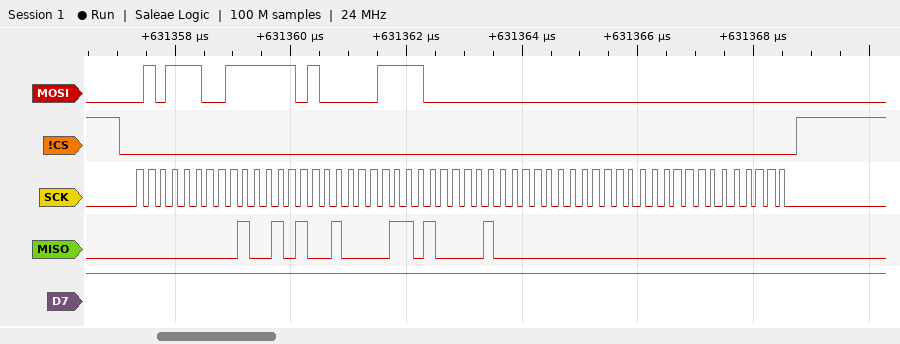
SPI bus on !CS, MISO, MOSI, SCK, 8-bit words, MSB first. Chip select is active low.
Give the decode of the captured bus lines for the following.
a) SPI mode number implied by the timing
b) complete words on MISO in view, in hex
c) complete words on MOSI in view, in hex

0
00, 4A, 43, 42, 00, 00, 00
5C, FD, 07, 80, 00, 00, 00
